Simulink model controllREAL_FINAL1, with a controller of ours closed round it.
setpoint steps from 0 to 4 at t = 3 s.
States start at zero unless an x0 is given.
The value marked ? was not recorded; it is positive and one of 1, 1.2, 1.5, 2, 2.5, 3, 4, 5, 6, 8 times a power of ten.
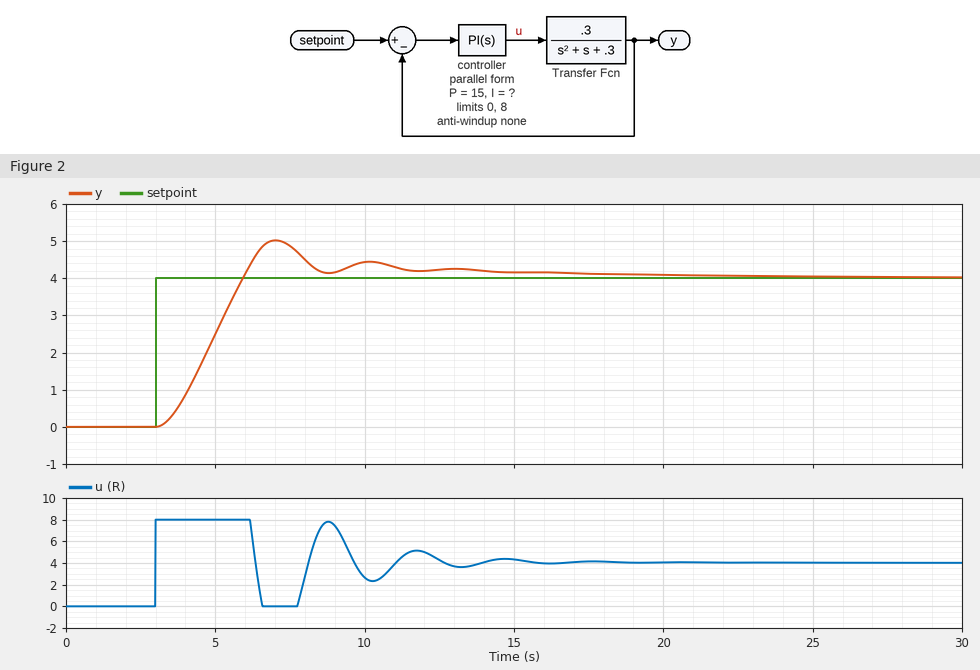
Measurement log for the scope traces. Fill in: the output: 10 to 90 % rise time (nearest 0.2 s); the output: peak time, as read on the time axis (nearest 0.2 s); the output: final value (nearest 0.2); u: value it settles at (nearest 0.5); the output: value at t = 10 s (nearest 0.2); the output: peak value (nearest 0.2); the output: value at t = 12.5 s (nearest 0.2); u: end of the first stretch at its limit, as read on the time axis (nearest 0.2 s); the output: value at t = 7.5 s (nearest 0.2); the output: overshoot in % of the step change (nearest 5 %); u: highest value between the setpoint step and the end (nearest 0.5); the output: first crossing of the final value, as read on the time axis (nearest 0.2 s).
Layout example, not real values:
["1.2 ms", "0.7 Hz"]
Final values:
["2.0 s", "7.0 s", "4.0", "4.0", "4.4", "5.0", "4.2", "6.2 s", "4.8", "25 %", "8.0", "6.0 s"]
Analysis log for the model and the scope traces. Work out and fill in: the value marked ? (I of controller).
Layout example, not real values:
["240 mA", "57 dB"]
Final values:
["2"]
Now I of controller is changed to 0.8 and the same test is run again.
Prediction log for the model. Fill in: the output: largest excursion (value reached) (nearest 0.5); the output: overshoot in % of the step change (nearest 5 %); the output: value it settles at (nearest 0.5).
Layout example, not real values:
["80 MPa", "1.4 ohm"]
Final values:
["4.5", "15 %", "4.0"]
